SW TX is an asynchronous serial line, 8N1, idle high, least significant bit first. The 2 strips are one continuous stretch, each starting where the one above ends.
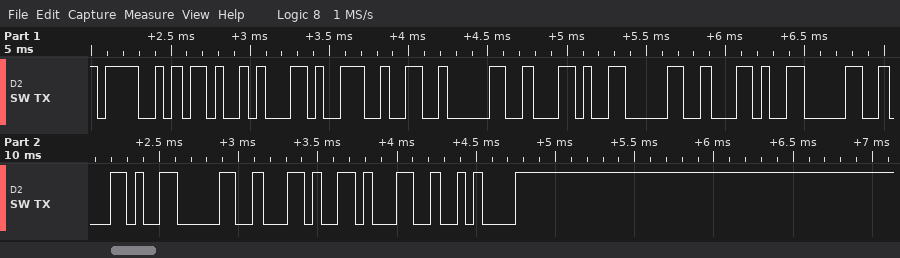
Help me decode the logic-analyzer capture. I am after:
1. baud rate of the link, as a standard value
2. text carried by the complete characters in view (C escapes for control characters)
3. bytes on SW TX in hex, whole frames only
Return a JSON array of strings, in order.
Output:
["19200 baud", "\"OK,20,0,0,0,1\\n\"", "0x4F 0x4B 0x2C 0x32 0x30 0x2C 0x30 0x2C 0x30 0x2C 0x30 0x2C 0x31 0x0A"]
